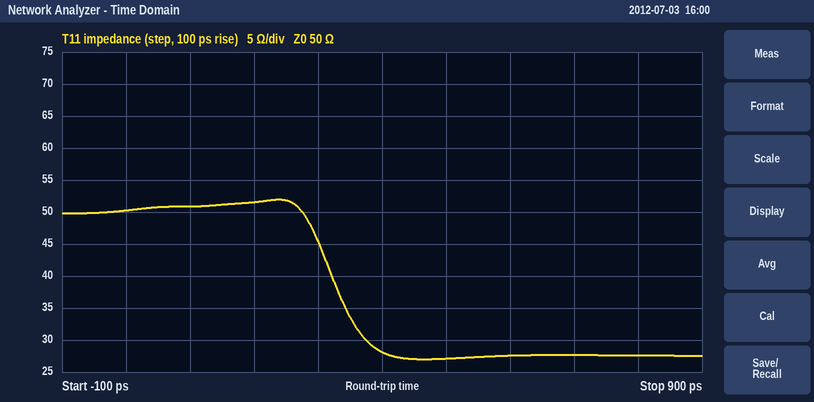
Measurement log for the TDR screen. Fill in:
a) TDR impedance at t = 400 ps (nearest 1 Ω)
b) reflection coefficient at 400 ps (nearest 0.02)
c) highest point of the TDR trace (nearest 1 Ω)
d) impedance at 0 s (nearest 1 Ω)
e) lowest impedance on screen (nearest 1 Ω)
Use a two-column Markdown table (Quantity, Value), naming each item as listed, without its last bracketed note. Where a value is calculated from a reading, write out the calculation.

| Quantity | Value |
|---|---|
| TDR impedance at t = 400 ps | 28 Ω |
| reflection coefficient at 400 ps | (28 − 50)/(28 + 50) ≈ -0.28 |
| highest point of the TDR trace | 52 Ω |
| impedance at 0 s | 50 Ω |
| lowest impedance on screen | 27 Ω |
